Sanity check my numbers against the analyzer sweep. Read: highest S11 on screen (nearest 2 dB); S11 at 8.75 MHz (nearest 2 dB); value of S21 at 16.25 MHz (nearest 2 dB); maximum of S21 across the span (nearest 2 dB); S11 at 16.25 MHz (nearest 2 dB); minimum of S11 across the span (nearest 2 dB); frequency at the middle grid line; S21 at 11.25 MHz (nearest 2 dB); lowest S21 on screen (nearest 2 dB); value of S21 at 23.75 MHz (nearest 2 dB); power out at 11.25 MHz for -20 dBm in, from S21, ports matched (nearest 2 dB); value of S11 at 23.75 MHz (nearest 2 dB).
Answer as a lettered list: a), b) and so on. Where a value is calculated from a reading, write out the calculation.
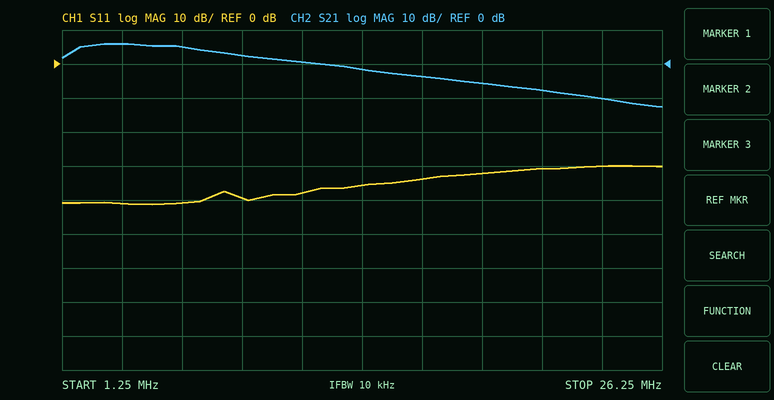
a) -30 dB
b) -40 dB
c) -4 dB
d) 6 dB
e) -34 dB
f) -42 dB
g) 13.75 MHz
h) 0 dB
i) -12 dB
j) -10 dB
k) -20 dBm + (0 dB) = -20 dBm
l) -30 dB
